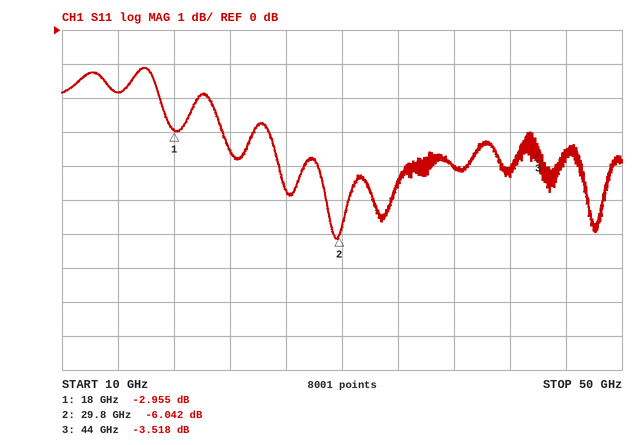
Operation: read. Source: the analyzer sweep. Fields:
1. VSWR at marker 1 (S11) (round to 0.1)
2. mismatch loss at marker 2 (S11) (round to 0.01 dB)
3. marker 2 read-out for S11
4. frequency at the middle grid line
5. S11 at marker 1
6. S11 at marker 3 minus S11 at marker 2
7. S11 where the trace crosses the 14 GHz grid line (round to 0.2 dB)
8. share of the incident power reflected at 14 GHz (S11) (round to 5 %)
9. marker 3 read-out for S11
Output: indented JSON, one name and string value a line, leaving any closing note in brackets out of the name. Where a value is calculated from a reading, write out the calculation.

{
  "VSWR at marker 1 (S11)": "(1 + 0.7116)/(1 − 0.7116) ≈ 5.9",
  "mismatch loss at marker 2 (S11)": "−10 log10(1 − 10^(-6.042/10)) ≈ 1.24 dB",
  "marker 2 read-out for S11": "-6.042 dB",
  "frequency at the middle grid line": "30 GHz",
  "S11 at marker 1": "-2.955 dB",
  "S11 at marker 3 minus S11 at marker 2": "-3.518 − (-6.042) = 2.524 dB",
  "S11 where the trace crosses the 14 GHz grid line": "-1.8 dB",
  "share of the incident power reflected at 14 GHz (S11)": "10^(-1.8/10) ≈ 66.1 %, so 65 % to the nearest 5 %",
  "marker 3 read-out for S11": "-3.518 dB"
}
